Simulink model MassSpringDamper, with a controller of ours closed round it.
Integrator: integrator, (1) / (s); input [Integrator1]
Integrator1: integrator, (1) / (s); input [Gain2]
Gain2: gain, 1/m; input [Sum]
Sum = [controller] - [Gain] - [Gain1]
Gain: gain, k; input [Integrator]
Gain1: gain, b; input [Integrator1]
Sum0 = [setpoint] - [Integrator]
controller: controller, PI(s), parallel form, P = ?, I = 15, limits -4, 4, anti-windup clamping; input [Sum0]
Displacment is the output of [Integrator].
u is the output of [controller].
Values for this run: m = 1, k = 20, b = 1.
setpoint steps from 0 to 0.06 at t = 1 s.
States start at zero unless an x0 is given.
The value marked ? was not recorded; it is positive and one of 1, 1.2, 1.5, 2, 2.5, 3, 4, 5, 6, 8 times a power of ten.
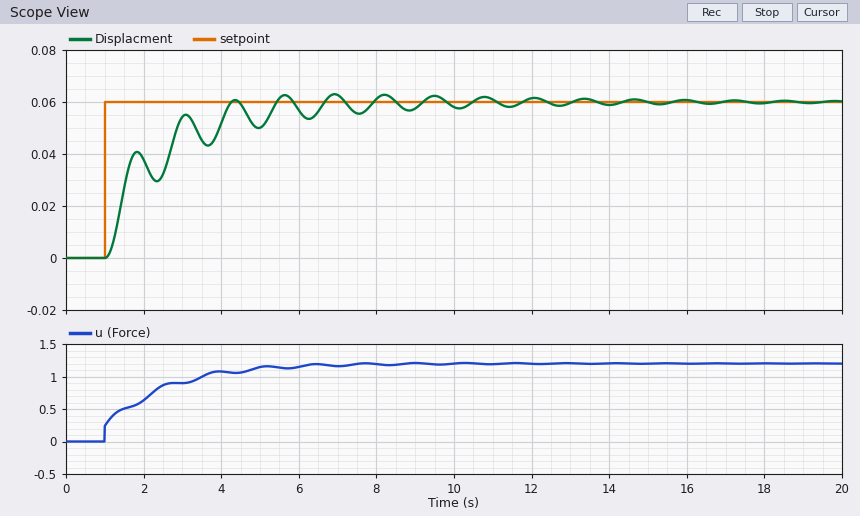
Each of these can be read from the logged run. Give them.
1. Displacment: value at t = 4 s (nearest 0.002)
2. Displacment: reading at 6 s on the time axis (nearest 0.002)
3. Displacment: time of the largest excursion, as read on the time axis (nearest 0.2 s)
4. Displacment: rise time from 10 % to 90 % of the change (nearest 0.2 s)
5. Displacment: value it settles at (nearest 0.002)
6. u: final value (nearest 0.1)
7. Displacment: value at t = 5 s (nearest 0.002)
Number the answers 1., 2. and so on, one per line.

1. 0.052
2. 0.056
3. 7.0 s
4. 1.8 s
5. 0.060
6. 1.2
7. 0.050
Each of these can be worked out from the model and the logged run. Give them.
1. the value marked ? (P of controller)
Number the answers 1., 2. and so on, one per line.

1. 4
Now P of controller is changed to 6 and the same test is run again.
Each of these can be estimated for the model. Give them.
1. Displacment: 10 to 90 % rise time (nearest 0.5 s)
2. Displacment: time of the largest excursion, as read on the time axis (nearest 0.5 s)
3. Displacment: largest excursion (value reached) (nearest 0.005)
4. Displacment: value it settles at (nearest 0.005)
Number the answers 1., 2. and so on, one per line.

1. 1.5 s
2. 6.5 s
3. 0.065
4. 0.060
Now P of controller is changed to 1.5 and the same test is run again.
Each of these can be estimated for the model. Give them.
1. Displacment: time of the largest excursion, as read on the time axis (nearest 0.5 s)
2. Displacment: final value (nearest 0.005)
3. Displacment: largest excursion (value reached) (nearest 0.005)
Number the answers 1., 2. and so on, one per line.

1. 7.5 s
2. 0.060
3. 0.065
